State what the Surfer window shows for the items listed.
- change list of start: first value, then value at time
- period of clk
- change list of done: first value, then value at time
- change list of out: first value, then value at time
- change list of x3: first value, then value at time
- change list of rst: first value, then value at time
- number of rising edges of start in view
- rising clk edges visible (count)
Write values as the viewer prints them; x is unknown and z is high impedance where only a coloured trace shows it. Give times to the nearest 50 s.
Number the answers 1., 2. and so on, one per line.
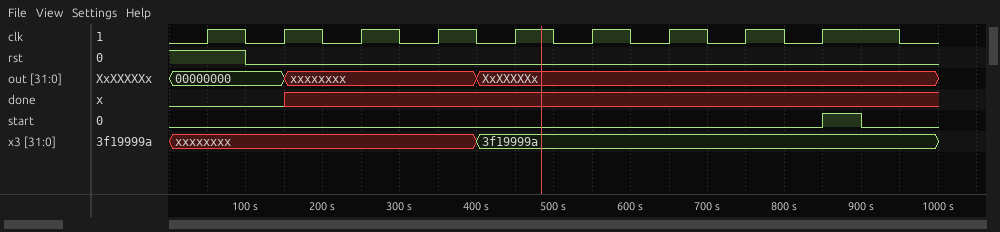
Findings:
1. 0, 1 at 850 s, 0 at 900 s
2. 100 s
3. 0, x at 150 s
4. 00000000, xxxxxxxx at 150 s, XxXXXXXx at 400 s
5. xxxxxxxx, 3f19999a at 400 s
6. 1, 0 at 100 s
7. 1
8. 9
